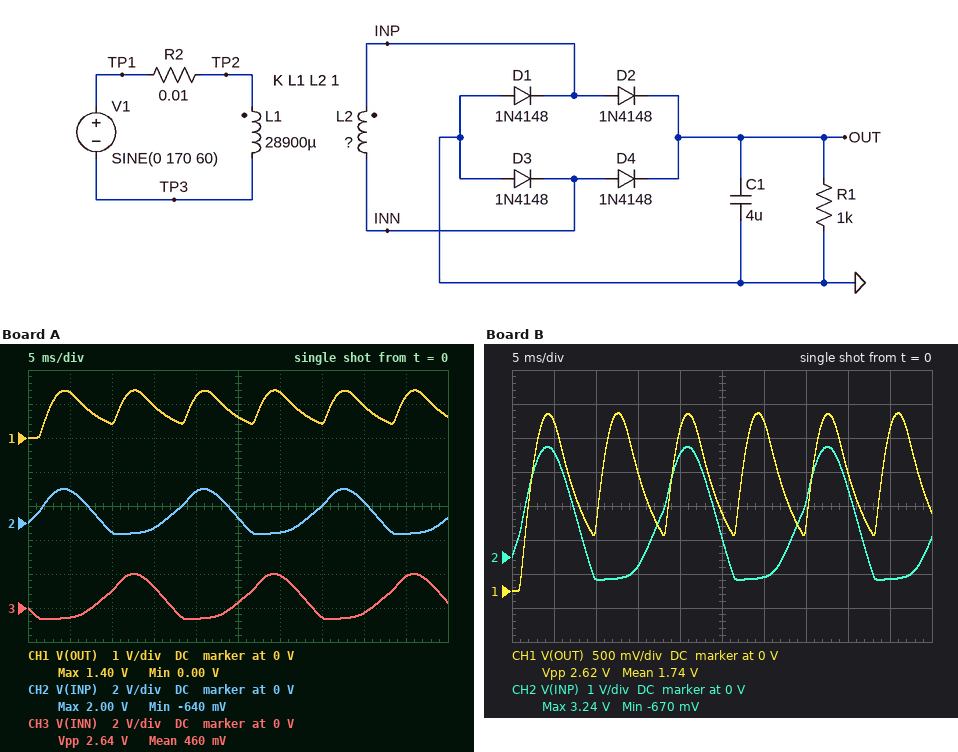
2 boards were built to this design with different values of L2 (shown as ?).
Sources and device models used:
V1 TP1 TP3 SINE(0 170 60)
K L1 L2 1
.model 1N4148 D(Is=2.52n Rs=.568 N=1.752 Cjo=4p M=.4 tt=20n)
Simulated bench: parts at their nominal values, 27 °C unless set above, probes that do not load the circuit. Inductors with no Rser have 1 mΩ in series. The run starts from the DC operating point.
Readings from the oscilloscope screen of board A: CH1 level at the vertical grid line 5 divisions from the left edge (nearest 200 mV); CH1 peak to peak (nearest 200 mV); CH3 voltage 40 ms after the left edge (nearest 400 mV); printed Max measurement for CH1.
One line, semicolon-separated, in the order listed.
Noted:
600 mV; 1.4 V; -400 mV; 1.40 V
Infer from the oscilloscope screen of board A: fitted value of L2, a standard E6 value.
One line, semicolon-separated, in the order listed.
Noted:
6.8 µH
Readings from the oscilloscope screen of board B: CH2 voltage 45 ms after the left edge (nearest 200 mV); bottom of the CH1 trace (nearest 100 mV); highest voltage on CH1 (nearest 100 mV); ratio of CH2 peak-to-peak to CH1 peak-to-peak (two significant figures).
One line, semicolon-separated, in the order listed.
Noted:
-600 mV; 0 V; 2.6 V; 1.5
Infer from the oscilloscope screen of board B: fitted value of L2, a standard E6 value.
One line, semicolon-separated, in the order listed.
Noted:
15 µH
